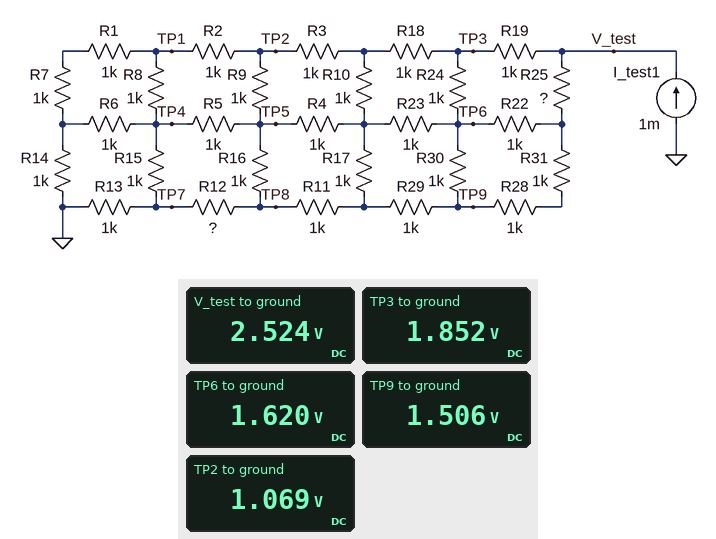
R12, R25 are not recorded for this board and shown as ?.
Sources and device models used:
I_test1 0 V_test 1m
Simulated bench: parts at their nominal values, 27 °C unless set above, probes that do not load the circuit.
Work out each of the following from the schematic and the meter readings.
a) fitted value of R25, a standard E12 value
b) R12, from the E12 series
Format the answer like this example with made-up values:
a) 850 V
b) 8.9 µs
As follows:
a) 2.2 kΩ
b) 820 Ω
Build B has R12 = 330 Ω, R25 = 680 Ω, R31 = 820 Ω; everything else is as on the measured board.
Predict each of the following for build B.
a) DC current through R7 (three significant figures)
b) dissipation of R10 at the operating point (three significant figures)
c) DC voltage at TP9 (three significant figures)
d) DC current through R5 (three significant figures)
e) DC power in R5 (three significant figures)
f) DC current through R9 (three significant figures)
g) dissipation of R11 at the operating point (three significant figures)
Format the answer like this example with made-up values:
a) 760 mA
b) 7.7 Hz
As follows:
a) 162 µA
b) 4.61 µW
c) 1.44 V
d) 243 µA
e) 58.9 µW
f) 71.2 µA
g) 143 µW
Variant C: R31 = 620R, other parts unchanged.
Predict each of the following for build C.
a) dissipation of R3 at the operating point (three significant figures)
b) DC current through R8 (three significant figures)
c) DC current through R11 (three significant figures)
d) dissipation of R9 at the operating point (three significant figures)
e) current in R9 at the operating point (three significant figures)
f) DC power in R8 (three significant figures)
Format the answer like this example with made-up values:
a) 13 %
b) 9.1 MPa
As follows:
a) 118 µW
b) 95.9 µA
c) 337 µA
d) 4.79 µW
e) 69.2 µA
f) 9.20 µW
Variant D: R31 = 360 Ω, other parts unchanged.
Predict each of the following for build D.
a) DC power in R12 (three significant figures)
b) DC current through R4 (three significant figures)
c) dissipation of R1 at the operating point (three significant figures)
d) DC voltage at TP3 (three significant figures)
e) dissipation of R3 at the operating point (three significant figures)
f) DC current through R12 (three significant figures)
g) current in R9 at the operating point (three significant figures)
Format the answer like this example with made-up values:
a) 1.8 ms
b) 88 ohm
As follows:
a) 149 µW
b) 319 µA
c) 31.6 µW
d) 1.84 V
e) 117 µW
f) 426 µA
g) 68.6 µA
